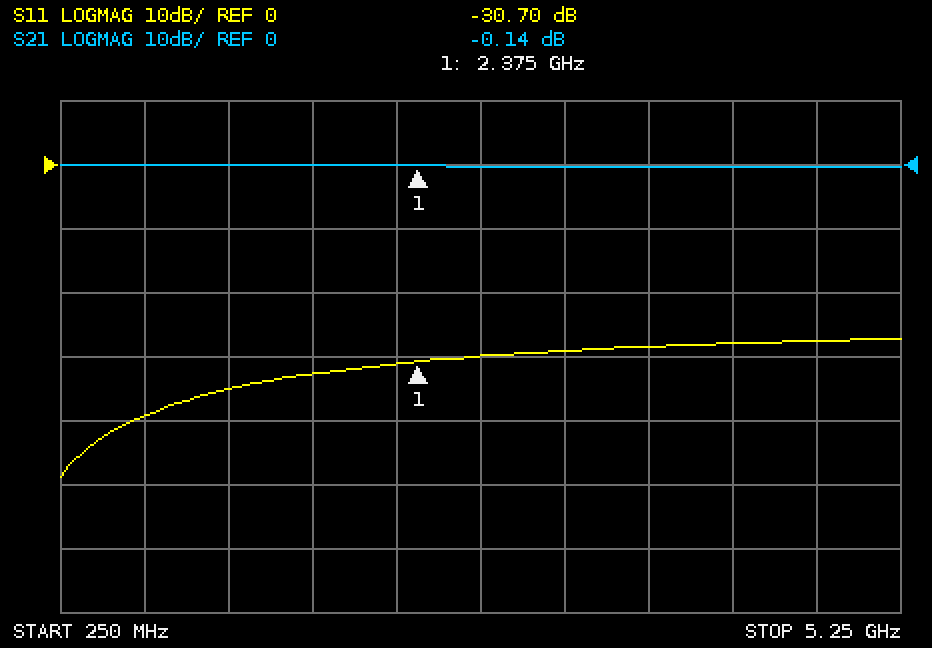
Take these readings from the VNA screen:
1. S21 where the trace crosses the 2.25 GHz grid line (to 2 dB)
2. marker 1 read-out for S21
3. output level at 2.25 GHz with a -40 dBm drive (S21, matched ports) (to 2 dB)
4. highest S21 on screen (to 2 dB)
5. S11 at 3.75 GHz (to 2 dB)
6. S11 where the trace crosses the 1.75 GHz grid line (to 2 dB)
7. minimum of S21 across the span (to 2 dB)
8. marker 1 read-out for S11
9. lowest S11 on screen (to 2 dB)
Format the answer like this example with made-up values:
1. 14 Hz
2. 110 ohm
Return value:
1. 0 dB
2. -0.14 dB
3. -40 dBm
4. 0 dB
5. -28 dB
6. -32 dB
7. 0 dB
8. -30.70 dB
9. -48 dB
